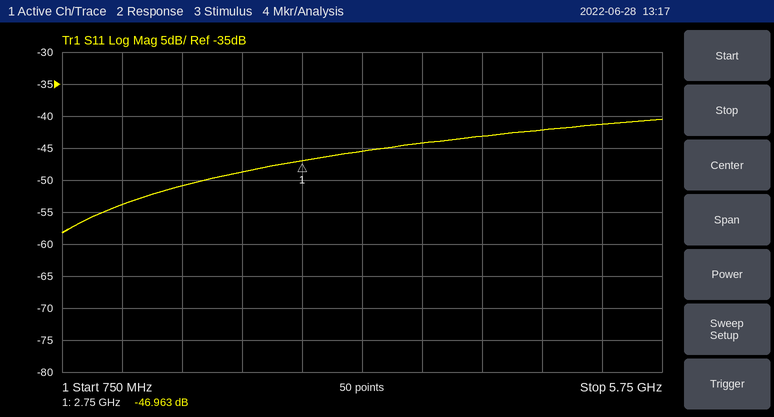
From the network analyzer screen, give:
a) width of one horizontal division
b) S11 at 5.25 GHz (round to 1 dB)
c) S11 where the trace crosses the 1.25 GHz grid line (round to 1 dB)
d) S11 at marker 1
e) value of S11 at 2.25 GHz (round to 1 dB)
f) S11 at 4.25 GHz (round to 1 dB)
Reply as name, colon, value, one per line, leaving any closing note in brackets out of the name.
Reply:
width of one horizontal division: 500 MHz
S11 at 5.25 GHz: -41 dB
S11 where the trace crosses the 1.25 GHz grid line: -54 dB
S11 at marker 1: -46.963 dB
value of S11 at 2.25 GHz: -49 dB
S11 at 4.25 GHz: -43 dB
